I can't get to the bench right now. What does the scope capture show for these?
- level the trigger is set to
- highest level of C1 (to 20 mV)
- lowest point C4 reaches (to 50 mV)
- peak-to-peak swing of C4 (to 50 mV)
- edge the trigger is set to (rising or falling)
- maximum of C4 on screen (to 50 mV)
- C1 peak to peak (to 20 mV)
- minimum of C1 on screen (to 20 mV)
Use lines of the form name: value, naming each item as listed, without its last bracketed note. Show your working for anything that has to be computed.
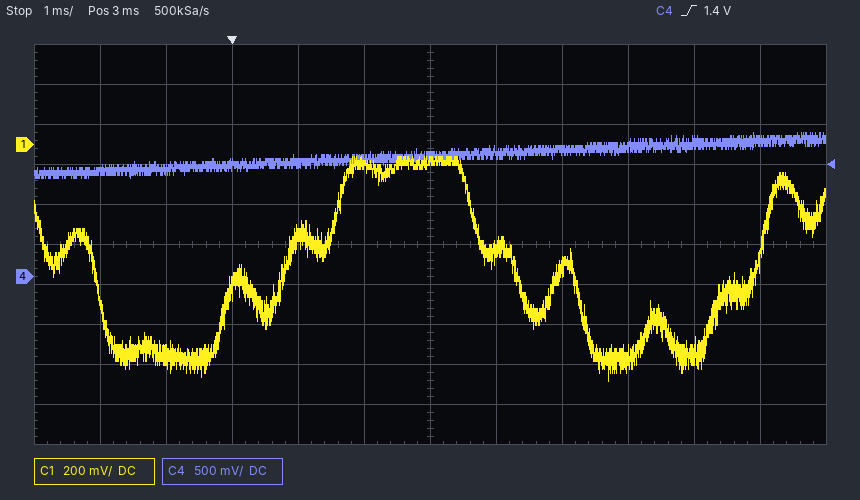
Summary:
level the trigger is set to: 1.4 V
highest level of C1: -60 mV
lowest point C4 reaches: 1.25 V
peak-to-peak swing of C4: 1.80 V − (1.25 V) = 550 mV
edge the trigger is set to: rising
maximum of C4 on screen: 1.80 V
C1 peak to peak: -60 mV − (-1.18 V) = 1.12 V
minimum of C1 on screen: -1.18 V
